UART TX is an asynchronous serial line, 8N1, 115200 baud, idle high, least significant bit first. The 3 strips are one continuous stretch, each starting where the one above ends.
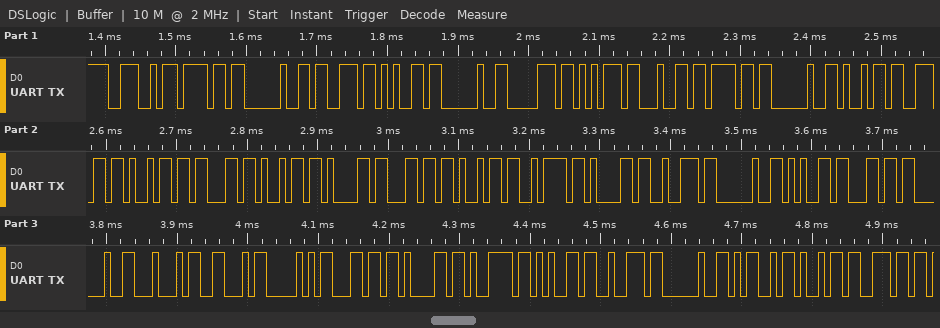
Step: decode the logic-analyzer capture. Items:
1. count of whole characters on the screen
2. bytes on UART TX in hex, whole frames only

38
4E 6F 20 73 65 20 70 75 64 6F 20 69 6E 69 63 69 61 6C 69 7A 61 72 20 65 6C 20 44 46 50 6C 61 79 65 72 20 4D 69 6E
